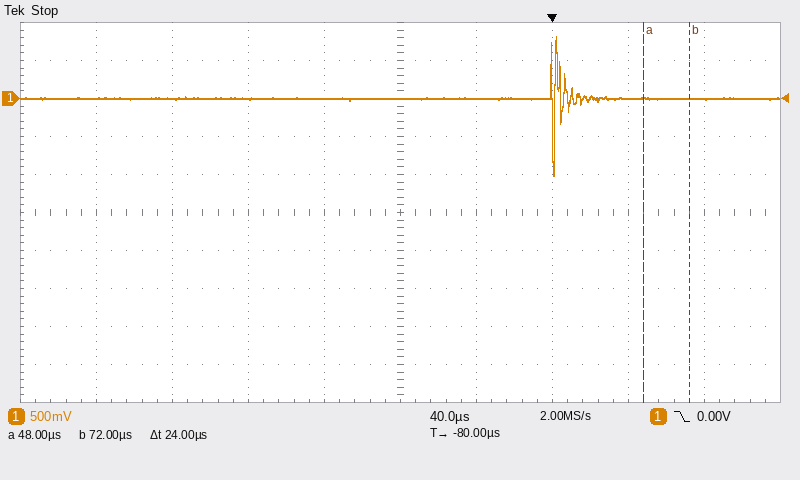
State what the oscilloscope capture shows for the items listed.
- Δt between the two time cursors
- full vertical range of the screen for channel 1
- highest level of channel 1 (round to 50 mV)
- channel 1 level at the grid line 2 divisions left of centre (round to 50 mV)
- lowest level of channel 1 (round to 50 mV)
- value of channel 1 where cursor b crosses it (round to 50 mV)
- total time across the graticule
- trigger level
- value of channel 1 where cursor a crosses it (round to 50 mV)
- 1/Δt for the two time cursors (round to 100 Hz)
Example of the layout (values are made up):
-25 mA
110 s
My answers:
24 µs
5 V
800 mV
0 mV
-1.00 V
0 mV
400 µs
0.00 V
0 mV
41.7 kHz
